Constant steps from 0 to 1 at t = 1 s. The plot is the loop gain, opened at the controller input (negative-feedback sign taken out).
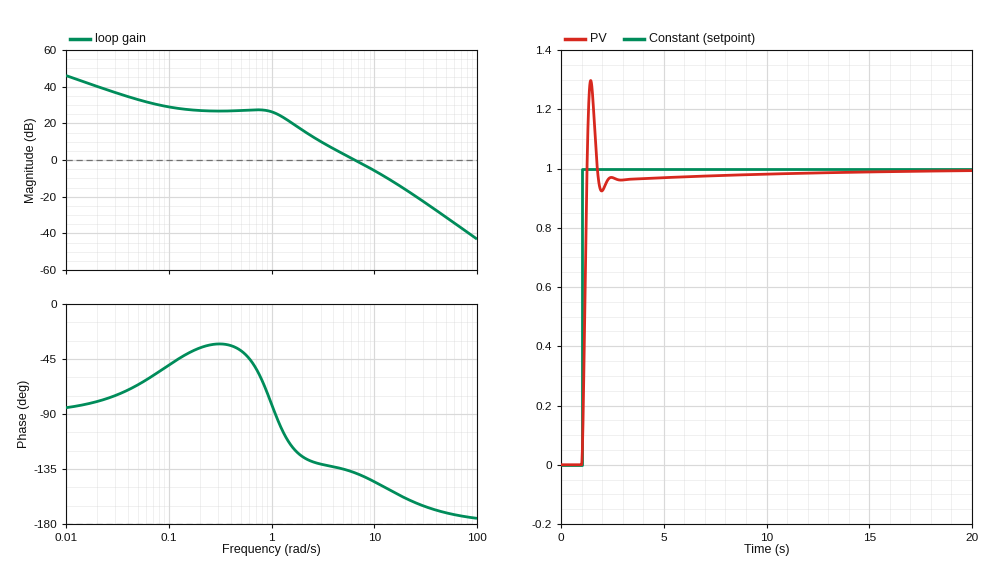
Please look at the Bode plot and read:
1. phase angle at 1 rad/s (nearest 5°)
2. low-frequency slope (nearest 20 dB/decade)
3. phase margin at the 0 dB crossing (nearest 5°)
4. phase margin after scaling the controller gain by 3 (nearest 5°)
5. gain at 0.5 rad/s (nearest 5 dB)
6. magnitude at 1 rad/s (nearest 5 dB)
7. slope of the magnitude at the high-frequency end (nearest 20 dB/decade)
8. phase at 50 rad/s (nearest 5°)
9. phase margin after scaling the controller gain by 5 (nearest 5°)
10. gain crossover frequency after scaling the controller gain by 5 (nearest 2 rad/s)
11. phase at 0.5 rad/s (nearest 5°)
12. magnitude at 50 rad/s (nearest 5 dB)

-80°
-20 dB/decade
40°
30°
25 dB
25 dB
-40 dB/decade
-170°
25°
18 rad/s
-40°
-30 dB
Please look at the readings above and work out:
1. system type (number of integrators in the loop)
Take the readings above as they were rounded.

1
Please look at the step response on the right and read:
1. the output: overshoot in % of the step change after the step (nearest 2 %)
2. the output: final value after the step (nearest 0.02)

30 %
1.00
